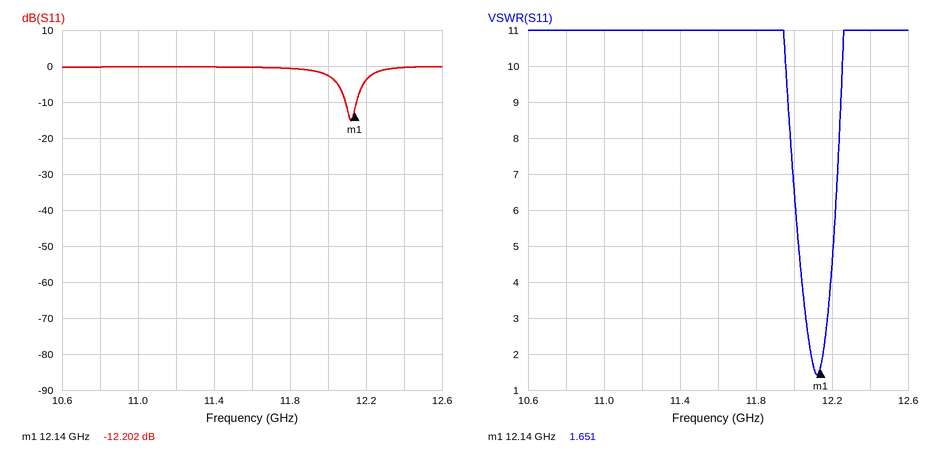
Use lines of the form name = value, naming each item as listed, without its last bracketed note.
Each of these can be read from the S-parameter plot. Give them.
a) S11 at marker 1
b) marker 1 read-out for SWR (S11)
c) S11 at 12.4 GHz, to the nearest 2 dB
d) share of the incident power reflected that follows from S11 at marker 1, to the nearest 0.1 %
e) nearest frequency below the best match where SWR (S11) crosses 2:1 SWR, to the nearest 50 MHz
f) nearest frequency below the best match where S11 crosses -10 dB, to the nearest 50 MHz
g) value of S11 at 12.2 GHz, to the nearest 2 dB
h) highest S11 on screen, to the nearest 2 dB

S11 at marker 1 = -12.202 dB
marker 1 read-out for SWR = 1.651
S11 at 12.4 GHz, to the nearest 2 dB = 0 dB
share of the incident power reflected that follows from S11 at marker 1, to the nearest 0.1 % = 6.0 %
nearest frequency below the best match where SWR (S11) crosses 2:1 SWR, to the nearest 50 MHz = 12.10 GHz
nearest frequency below the best match where S11 crosses -10 dB, to the nearest 50 MHz = 12.10 GHz
value of S11 at 12.2 GHz, to the nearest 2 dB = -4 dB
highest S11 on screen, to the nearest 2 dB = 0 dB
